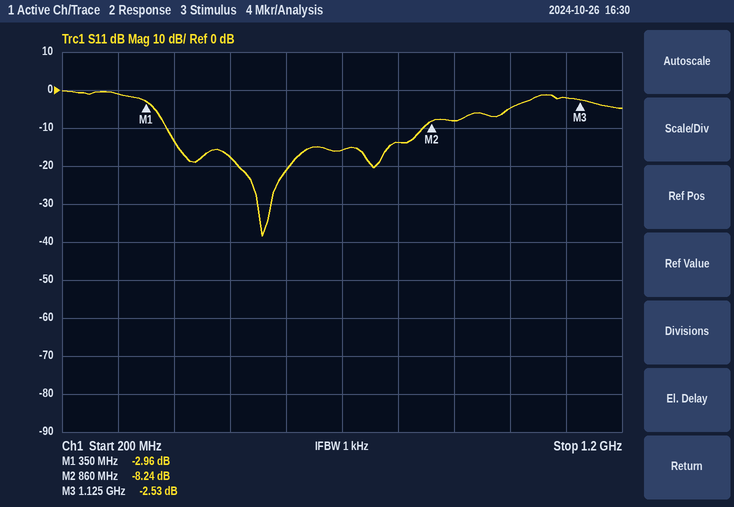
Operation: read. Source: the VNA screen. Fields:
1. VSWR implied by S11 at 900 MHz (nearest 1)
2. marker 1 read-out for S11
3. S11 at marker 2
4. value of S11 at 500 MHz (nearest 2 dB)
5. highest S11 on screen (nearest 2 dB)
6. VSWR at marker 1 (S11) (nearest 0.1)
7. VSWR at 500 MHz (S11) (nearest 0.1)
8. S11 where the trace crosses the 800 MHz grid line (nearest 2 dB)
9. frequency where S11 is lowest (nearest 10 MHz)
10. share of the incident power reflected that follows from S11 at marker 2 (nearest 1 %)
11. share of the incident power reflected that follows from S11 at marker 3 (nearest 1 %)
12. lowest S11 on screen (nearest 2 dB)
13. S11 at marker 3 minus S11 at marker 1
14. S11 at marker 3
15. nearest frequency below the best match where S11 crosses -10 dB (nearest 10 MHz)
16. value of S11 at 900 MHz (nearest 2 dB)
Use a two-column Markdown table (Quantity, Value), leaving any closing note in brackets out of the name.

| Quantity | Value |
|---|---|
| VSWR implied by S11 at 900 MHz | 2 |
| marker 1 read-out for S11 | -2.96 dB |
| S11 at marker 2 | -8.24 dB |
| value of S11 at 500 MHz | -18 dB |
| highest S11 on screen | 0 dB |
| VSWR at marker 1 (S11) | 5.9 |
| VSWR at 500 MHz (S11) | 1.3 |
| S11 where the trace crosses the 800 MHz grid line | -14 dB |
| frequency where S11 is lowest | 560 MHz |
| share of the incident power reflected that follows from S11 at marker 2 | 15 % |
| share of the incident power reflected that follows from S11 at marker 3 | 56 % |
| lowest S11 on screen | -38 dB |
| S11 at marker 3 minus S11 at marker 1 | 0.43 dB |
| S11 at marker 3 | -2.53 dB |
| nearest frequency below the best match where S11 crosses -10 dB | 390 MHz |
| value of S11 at 900 MHz | -8 dB |
